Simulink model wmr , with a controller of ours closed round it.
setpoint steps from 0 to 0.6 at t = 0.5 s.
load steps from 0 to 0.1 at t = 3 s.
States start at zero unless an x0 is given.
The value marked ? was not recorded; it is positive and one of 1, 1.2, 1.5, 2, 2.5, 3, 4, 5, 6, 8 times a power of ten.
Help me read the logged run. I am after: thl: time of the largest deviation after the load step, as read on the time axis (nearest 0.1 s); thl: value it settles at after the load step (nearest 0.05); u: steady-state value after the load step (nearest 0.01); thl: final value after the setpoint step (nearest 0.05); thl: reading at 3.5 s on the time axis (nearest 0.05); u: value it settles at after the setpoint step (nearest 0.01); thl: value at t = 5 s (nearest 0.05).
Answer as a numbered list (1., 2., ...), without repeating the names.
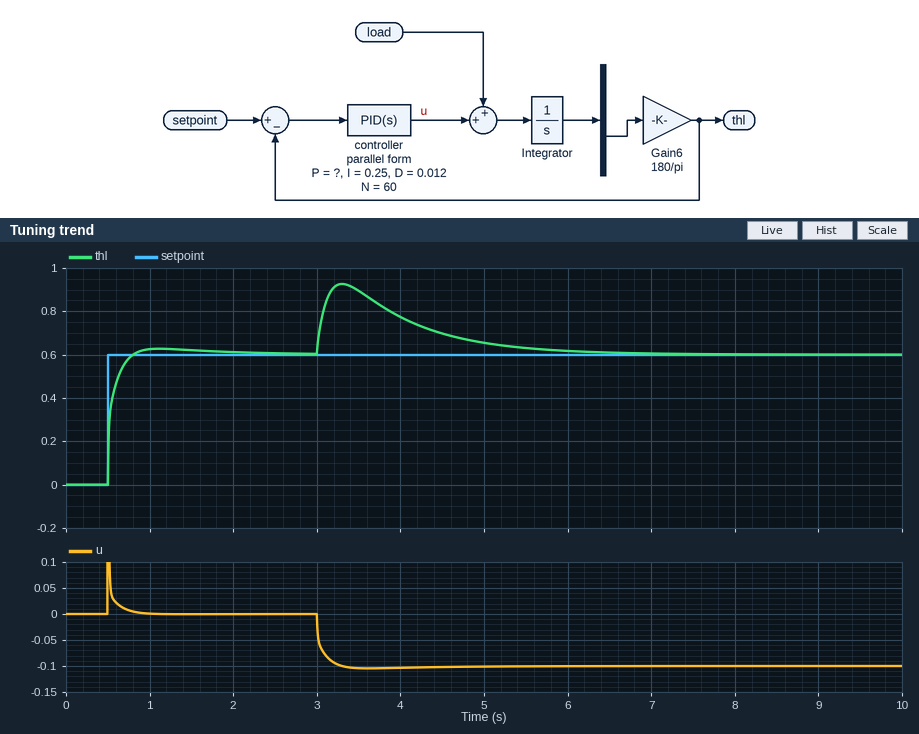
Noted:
1. 3.3 s
2. 0.60
3. -0.10
4. 0.60
5. 0.90
6. 0.00
7. 0.65
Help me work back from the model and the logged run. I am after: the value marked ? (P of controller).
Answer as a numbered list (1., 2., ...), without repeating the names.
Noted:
1. 0.25
